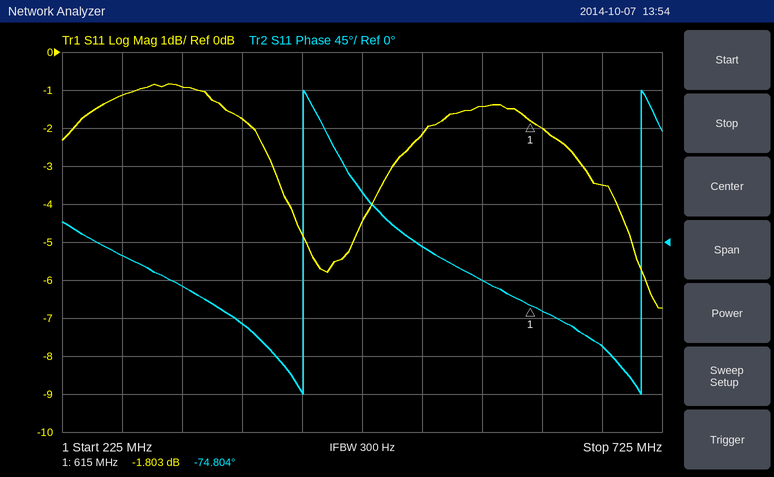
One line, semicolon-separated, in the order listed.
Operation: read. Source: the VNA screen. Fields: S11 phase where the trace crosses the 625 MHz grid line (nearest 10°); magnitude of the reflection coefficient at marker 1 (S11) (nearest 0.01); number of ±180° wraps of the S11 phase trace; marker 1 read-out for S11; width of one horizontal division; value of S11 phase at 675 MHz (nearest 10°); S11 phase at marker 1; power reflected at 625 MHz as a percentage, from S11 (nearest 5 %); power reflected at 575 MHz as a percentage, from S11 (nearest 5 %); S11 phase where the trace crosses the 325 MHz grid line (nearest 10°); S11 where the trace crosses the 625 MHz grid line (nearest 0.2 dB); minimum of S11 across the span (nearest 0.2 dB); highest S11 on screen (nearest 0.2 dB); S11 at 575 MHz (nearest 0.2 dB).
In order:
-80°; 0.81; 2; -1.803 dB; 50 MHz; -120°; -74.804°; 65 %; 70 %; -50°; -2.0 dB; -6.8 dB; -0.8 dB; -1.4 dB
